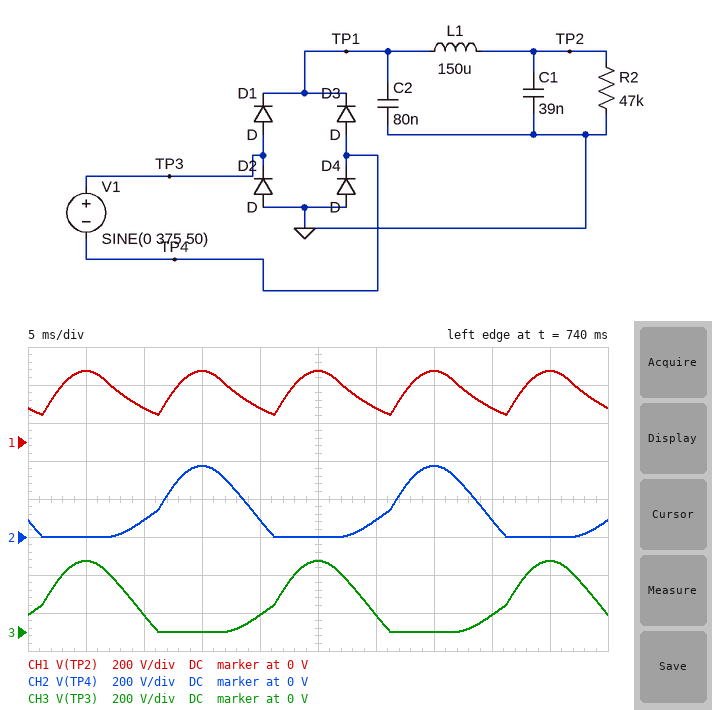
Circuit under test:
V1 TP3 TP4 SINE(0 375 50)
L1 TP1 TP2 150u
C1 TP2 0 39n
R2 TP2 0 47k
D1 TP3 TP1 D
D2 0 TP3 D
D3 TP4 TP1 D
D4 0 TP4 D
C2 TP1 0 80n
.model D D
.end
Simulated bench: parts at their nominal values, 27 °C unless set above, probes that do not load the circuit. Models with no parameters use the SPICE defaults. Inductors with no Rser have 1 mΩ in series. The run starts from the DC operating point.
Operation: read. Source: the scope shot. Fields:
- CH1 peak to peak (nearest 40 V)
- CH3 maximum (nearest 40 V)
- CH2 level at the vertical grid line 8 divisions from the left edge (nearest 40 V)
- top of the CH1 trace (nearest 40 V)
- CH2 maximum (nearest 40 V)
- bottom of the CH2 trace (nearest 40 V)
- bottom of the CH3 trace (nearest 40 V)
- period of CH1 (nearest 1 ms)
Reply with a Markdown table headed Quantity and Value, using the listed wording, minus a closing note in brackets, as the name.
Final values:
| Quantity | Value |
|---|---|
| CH1 peak to peak | 240 V |
| CH3 maximum | 360 V |
| CH2 level at the vertical grid line 8 divisions from the left edge | 80 V |
| top of the CH1 trace | 360 V |
| CH2 maximum | 360 V |
| bottom of the CH2 trace | 0 V |
| bottom of the CH3 trace | 0 V |
| period of CH1 | 10 ms |
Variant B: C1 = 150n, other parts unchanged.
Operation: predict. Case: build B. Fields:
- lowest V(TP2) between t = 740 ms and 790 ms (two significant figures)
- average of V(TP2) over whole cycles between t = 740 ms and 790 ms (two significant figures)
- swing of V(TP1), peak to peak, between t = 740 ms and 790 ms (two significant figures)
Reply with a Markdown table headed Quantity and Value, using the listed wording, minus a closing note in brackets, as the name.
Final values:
| Quantity | Value |
|---|---|
| lowest V(TP2) between t = 740 ms and 790 ms | 210 V |
| average of V(TP2) over whole cycles between t = 740 ms and 790 ms | 300 V |
| swing of V(TP1), peak to peak, between t = 740 ms and 790 ms | 170 V |
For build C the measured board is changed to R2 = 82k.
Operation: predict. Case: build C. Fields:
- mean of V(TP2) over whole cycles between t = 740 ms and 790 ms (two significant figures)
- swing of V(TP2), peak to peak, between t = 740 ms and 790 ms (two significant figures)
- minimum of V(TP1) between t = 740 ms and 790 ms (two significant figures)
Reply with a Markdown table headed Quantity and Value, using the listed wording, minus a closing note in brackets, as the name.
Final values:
| Quantity | Value |
|---|---|
| mean of V(TP2) over whole cycles between t = 740 ms and 790 ms | 290 V |
| swing of V(TP2), peak to peak, between t = 740 ms and 790 ms | 180 V |
| minimum of V(TP1) between t = 740 ms and 790 ms | 200 V |
